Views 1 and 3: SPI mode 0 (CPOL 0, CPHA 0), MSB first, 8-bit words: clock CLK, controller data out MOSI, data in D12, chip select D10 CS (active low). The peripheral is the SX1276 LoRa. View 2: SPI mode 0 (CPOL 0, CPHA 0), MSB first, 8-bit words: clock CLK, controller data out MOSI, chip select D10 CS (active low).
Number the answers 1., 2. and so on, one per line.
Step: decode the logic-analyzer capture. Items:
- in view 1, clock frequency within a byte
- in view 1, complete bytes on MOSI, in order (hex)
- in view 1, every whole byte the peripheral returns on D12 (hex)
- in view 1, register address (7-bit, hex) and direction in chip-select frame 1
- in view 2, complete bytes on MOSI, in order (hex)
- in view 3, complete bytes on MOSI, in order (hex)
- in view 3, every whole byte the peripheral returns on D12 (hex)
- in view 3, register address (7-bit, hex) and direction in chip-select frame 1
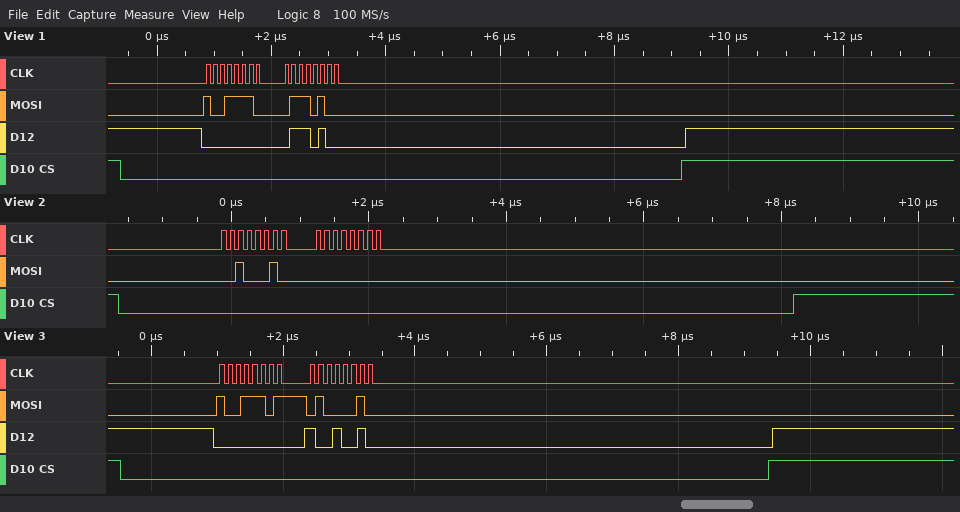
1. 8 MHz
2. 9E 74
3. 00 74
4. 0x1E write
5. 22 00
6. 9D 42
7. 00 92
8. 0x1D write
